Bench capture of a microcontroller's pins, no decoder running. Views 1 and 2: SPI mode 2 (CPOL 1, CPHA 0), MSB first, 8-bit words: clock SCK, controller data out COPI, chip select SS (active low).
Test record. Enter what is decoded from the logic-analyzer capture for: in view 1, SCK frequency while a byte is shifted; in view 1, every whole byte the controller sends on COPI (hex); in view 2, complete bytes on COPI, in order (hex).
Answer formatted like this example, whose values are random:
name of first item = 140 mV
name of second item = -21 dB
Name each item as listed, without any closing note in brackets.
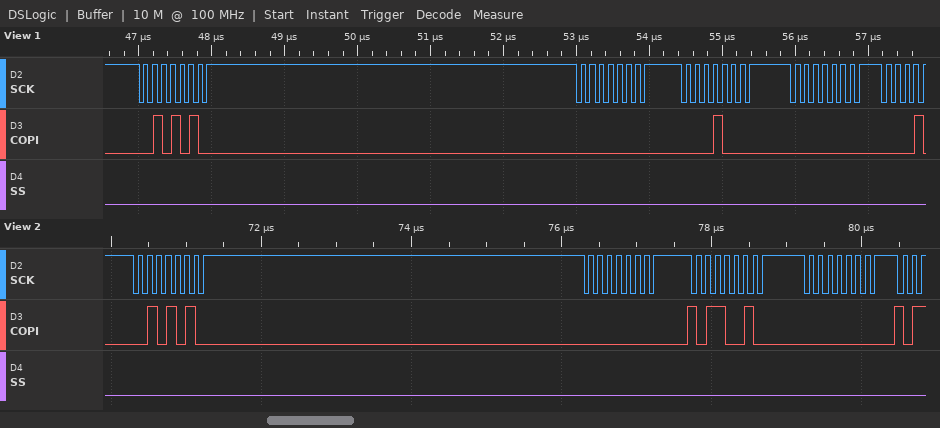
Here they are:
in view 1, SCK frequency while a byte is shifted = 8 MHz
in view 1, every whole byte the controller sends on COPI = 2A 00 08 00
in view 2, complete bytes on COPI, in order = 2A 00 B2 00
